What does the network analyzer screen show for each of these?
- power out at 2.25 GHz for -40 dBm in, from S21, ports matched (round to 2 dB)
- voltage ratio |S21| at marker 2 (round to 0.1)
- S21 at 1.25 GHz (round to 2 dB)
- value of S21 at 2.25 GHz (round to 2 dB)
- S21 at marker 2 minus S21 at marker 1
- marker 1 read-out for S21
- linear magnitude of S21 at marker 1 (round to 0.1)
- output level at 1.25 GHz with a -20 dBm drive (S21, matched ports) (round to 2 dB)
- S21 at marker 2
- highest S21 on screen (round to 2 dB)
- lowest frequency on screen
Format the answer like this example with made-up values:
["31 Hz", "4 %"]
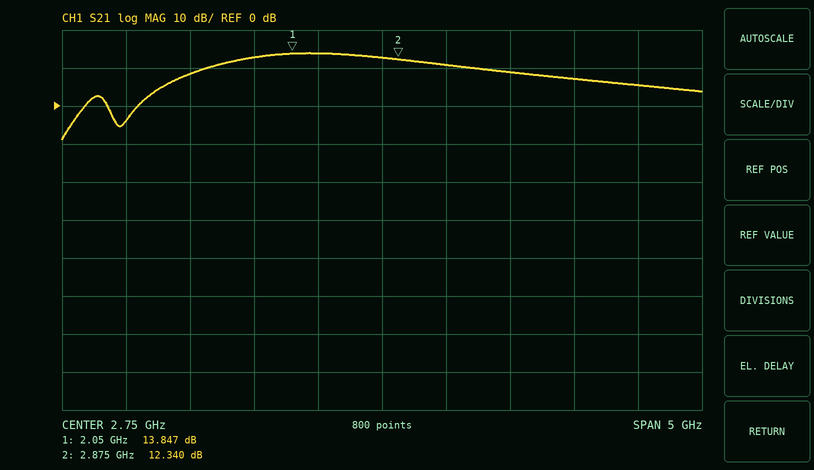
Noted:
["-26 dBm", "4.1", "8 dB", "14 dB", "-1.507 dB", "13.847 dB", "4.9", "-12 dBm", "12.340 dB", "14 dB", "250 MHz"]
